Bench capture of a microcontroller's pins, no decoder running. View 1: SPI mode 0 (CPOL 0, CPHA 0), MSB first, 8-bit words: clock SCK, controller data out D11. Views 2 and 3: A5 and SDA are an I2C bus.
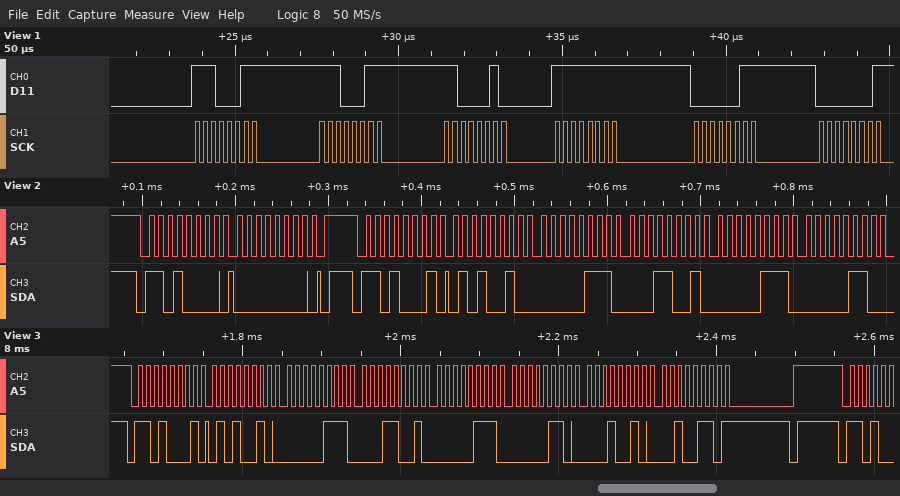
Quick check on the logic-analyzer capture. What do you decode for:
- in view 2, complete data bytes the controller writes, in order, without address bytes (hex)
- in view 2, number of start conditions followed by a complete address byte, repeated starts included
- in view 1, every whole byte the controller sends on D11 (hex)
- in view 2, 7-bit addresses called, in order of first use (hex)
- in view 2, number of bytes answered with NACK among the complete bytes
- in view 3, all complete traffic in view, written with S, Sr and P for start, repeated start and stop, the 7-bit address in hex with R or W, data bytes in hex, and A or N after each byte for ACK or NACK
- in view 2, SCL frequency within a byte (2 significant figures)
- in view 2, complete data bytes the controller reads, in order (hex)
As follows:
00
2
0xE3 0xE3 0xC2 0xFF 0x03 0x01
0x68
0
S 68R A 52 A 07 A 19 A 07 A 06 A 12 A 26 N P
100 kHz
52 07 19 07 06
